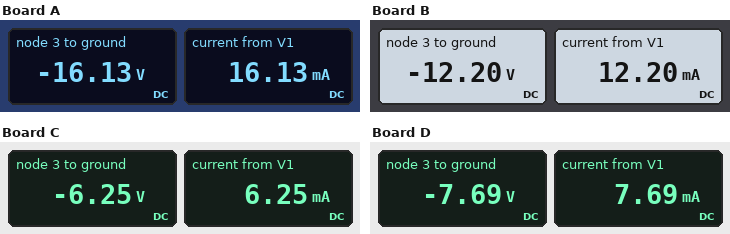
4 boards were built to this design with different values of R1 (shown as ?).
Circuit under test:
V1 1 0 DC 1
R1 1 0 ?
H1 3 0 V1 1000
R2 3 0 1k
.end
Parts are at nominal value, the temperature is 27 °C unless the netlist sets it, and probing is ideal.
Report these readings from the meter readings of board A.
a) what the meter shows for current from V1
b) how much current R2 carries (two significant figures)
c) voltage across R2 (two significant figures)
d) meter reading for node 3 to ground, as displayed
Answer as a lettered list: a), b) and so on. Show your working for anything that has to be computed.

a) 16.13 mA
b) (0 V - (-16.13 V)) / 1 kΩ = 16 mA
c) 0 V - (-16.13 V) = 16 V
d) -16.13 V
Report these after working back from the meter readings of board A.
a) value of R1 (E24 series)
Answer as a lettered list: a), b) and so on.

a) 62 Ω
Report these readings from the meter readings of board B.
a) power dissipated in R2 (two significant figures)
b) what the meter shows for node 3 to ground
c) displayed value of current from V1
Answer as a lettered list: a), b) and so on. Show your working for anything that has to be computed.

a) (0 V - (-12.2 V))^2 / 1 kΩ = 150 mW
b) -12.20 V
c) 12.20 mA
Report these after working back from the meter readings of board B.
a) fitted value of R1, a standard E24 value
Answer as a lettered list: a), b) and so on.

a) 82 Ω
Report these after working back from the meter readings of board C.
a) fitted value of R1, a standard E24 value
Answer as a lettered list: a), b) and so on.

a) 160 Ω
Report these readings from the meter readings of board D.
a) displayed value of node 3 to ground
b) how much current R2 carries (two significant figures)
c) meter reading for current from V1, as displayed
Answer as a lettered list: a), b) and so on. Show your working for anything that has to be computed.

a) -7.69 V
b) (0 V - (-7.69 V)) / 1 kΩ = 7.7 mA
c) 7.69 mA
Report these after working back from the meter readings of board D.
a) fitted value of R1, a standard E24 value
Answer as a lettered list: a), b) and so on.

a) 130 Ω
